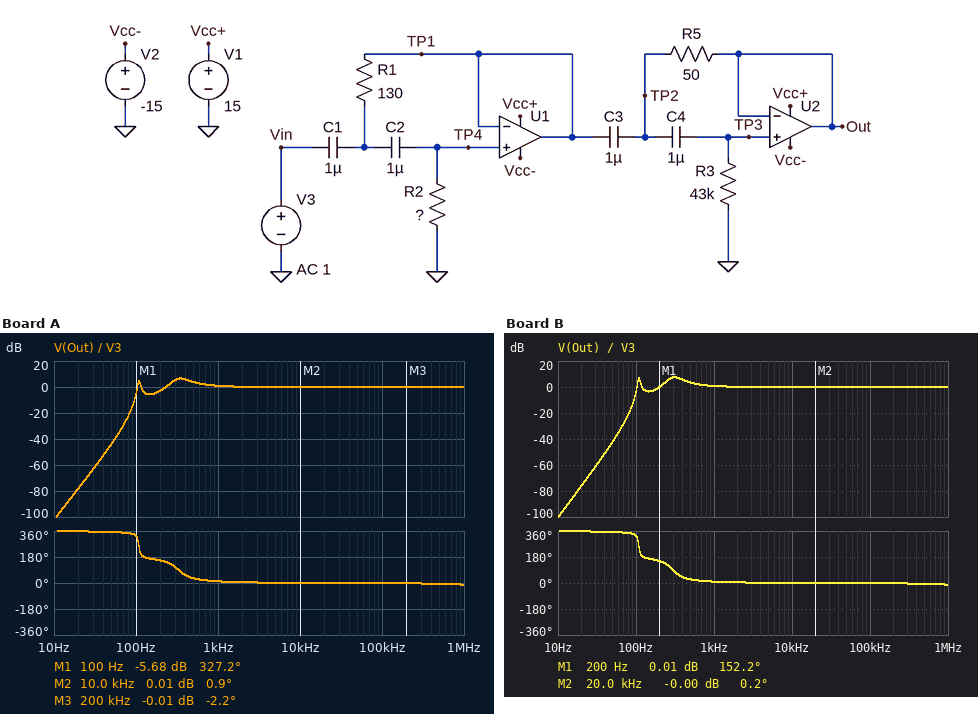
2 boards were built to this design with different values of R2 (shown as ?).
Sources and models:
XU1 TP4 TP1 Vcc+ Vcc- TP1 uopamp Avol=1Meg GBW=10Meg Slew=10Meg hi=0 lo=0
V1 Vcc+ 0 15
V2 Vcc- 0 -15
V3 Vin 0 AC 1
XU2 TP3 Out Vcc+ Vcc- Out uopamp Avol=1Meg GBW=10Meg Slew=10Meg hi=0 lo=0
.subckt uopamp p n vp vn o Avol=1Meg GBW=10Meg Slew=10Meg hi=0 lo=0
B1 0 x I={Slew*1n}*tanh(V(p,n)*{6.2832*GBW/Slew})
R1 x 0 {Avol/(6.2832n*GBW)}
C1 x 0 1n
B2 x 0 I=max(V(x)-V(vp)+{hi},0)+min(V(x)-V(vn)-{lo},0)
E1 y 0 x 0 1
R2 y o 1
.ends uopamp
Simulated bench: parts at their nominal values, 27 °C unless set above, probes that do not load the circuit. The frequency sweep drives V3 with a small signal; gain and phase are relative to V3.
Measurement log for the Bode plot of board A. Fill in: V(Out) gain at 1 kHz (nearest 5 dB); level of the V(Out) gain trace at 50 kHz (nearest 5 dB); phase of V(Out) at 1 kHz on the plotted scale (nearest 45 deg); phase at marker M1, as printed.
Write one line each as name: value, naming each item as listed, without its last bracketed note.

V(Out) gain at 1 kHz: 0 dB
level of the V(Out) gain trace at 50 kHz: 0 dB
phase of V(Out) at 1 kHz on the plotted scale: 0 deg
phase at marker M1, as printed: 327.2 deg
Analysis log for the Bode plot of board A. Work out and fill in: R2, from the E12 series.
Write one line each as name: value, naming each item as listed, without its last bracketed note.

R2, from the E12 series: 1.8 kΩ
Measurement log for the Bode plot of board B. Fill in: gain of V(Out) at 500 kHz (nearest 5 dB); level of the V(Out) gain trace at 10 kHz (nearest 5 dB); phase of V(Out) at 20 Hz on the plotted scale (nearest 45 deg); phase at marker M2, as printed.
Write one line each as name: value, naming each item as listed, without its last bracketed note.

gain of V(Out) at 500 kHz: 0 dB
level of the V(Out) gain trace at 10 kHz: 0 dB
phase of V(Out) at 20 Hz on the plotted scale: 360 deg
phase at marker M2, as printed: 0.2 deg
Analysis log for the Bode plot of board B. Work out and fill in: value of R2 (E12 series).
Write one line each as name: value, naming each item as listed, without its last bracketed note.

value of R2: 2.2 kΩ
